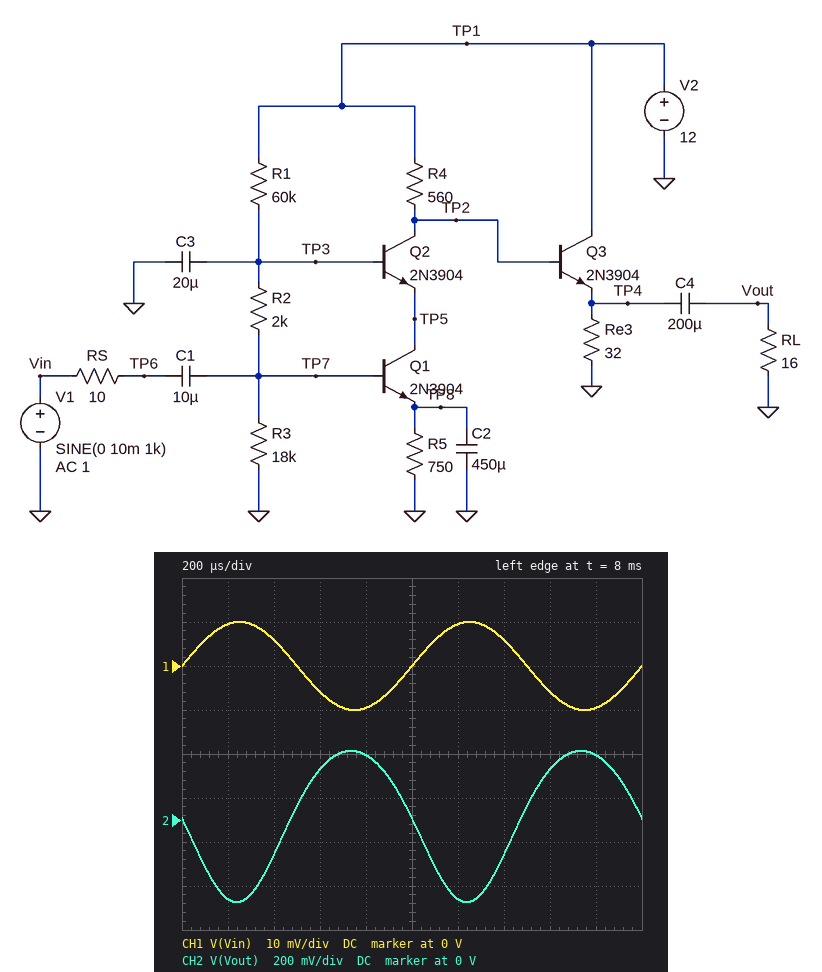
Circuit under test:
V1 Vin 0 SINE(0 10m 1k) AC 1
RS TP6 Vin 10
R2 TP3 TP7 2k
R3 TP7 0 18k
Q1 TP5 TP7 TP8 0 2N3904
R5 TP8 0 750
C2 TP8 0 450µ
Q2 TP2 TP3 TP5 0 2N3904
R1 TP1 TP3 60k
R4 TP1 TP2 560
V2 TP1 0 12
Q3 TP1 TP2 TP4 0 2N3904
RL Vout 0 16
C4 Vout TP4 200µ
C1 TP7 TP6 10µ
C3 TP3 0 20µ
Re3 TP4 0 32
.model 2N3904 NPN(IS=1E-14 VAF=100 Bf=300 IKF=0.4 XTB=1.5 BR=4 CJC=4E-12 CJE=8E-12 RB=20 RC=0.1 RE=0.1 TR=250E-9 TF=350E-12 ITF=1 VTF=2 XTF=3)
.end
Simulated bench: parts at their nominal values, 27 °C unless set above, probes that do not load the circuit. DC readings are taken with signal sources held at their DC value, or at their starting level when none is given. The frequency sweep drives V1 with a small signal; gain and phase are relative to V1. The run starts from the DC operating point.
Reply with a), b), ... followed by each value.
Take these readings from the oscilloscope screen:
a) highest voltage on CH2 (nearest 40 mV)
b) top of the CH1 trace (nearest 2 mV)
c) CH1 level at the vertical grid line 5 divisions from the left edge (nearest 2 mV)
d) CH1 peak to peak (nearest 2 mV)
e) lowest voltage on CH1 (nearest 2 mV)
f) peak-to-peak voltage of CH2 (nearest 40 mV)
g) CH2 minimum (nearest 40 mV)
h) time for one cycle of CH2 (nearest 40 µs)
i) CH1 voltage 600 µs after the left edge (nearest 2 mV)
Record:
a) 320 mV
b) 10 mV
c) 0 V
d) 20 mV
e) -10 mV
f) 680 mV
g) -360 mV
h) 1.00 ms
i) -6 mV
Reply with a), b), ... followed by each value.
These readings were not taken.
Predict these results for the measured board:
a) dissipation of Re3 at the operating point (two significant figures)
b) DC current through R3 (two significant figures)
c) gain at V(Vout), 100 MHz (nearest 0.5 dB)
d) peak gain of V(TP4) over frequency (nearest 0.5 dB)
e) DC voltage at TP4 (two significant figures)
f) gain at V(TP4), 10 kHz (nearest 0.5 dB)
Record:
a) 2.5 W
b) 140 µA
c) 4.5 dB
d) 31.0 dB
e) 8.9 V
f) 31.0 dB
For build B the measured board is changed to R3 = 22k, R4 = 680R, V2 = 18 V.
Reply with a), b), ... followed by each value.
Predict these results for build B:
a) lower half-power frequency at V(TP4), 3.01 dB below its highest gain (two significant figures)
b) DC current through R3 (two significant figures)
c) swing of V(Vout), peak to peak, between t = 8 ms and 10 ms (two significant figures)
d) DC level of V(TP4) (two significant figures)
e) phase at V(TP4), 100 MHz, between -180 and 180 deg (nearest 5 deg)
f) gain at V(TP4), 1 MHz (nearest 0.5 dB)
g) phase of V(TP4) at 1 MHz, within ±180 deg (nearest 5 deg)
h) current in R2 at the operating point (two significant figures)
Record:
a) 62 Hz
b) 190 µA
c) 1.4 V
d) 12 V
e) 30 deg
f) 37.0 dB
g) 170 deg
h) 210 µA
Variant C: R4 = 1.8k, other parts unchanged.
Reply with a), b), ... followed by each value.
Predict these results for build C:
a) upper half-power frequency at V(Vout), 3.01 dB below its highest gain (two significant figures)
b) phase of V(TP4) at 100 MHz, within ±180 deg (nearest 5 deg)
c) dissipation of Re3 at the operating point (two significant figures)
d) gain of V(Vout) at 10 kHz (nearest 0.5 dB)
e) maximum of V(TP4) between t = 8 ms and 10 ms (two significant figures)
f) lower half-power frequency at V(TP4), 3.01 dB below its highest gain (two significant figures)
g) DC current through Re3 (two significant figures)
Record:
a) 4.5 MHz
b) 35 deg
c) 950 mW
d) 38.0 dB
e) 6.2 V
f) 27 Hz
g) 170 mA
